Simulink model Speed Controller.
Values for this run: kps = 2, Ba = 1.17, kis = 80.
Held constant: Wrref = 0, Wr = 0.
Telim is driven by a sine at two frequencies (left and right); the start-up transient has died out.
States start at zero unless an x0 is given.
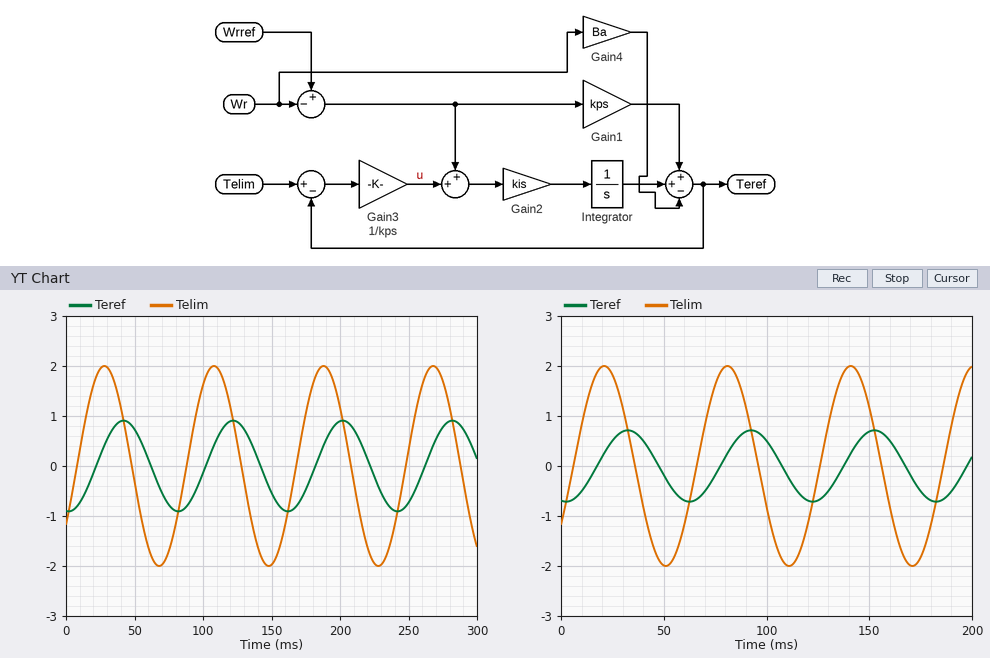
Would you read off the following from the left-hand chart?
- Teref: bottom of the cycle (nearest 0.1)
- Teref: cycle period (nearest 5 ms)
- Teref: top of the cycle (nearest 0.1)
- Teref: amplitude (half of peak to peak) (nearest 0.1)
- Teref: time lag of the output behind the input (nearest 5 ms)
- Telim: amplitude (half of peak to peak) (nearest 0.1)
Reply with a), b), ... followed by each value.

a) -0.9
b) 80 ms
c) 0.9
d) 0.9
e) 15 ms
f) 2.0
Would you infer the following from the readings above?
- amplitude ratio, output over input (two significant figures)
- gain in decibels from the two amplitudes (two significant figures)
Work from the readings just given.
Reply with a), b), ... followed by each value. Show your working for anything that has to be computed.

a) 0.9 / 2 = 0.45
b) 20 log10(0.9 / 2) = -6.9 dB
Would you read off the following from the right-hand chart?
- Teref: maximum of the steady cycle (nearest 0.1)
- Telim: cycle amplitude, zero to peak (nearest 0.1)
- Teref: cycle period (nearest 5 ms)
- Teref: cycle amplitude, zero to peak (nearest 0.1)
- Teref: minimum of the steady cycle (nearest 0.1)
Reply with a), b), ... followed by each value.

a) 0.7
b) 2.0
c) 60 ms
d) 0.7
e) -0.7
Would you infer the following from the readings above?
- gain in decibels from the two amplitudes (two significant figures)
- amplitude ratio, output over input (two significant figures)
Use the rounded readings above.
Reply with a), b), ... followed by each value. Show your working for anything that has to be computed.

a) 20 log10(0.7 / 2) = -9.1 dB
b) 0.7 / 2 = 0.35
